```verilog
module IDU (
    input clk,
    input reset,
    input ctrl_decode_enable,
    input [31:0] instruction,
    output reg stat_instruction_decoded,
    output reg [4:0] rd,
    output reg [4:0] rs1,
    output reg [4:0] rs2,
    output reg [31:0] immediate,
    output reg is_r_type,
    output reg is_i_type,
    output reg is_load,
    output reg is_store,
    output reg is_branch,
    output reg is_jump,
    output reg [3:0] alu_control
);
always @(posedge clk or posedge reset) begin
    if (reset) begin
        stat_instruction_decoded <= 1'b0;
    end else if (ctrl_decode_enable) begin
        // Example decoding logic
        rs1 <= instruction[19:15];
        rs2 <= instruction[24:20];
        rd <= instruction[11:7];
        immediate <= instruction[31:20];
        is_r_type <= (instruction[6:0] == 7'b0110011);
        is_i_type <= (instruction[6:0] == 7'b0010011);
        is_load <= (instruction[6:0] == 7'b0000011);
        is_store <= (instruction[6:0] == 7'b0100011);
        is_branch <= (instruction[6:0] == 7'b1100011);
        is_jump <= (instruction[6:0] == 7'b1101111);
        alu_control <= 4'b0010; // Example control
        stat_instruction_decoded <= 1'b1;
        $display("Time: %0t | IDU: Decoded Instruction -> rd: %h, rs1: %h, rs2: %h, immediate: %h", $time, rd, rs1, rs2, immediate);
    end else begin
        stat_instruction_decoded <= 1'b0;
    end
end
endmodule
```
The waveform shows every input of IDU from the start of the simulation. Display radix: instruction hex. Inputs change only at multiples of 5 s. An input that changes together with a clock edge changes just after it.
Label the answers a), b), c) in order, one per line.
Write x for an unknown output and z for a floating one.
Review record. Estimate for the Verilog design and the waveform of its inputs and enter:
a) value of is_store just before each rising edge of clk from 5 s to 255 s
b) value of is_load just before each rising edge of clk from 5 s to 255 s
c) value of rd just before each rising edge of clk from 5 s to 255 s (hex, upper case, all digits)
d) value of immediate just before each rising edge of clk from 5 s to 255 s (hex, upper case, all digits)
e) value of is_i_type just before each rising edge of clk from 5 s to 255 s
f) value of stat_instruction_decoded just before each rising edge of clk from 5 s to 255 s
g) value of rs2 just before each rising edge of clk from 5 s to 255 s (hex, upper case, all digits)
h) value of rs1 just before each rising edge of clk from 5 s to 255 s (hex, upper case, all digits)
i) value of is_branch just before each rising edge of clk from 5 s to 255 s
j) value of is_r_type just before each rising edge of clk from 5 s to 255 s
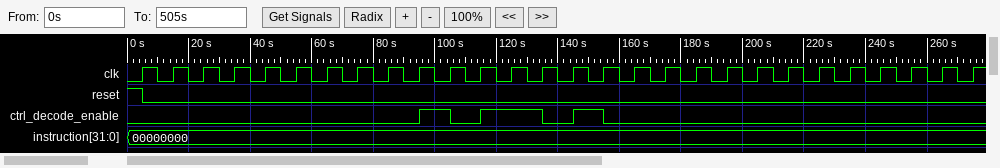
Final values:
a) x x x x x x x x x x x 0 0 0 0 0 0 0 0 0 0 0 0 0 0 0
b) x x x x x x x x x x x 0 0 0 0 0 0 0 0 0 0 0 0 0 0 0
c) x, x, x, x, x, x, x, x, x, x, x, 00, 00, 00, 00, 00, 00, 00, 00, 00, 00, 00, 00, 00, 00, 00
d) x, x, x, x, x, x, x, x, x, x, x, 00000000, 00000000, 00000000, 00000000, 00000000, 00000000, 00000000, 00000000, 00000000, 00000000, 00000000, 00000000, 00000000, 00000000, 00000000
e) x x x x x x x x x x x 0 0 0 0 0 0 0 0 0 0 0 0 0 0 0
f) 0 0 0 0 0 0 0 0 0 0 0 1 0 1 1 0 1 0 0 0 0 0 0 0 0 0
g) x, x, x, x, x, x, x, x, x, x, x, 00, 00, 00, 00, 00, 00, 00, 00, 00, 00, 00, 00, 00, 00, 00
h) x, x, x, x, x, x, x, x, x, x, x, 00, 00, 00, 00, 00, 00, 00, 00, 00, 00, 00, 00, 00, 00, 00
i) x x x x x x x x x x x 0 0 0 0 0 0 0 0 0 0 0 0 0 0 0
j) x x x x x x x x x x x 0 0 0 0 0 0 0 0 0 0 0 0 0 0 0
